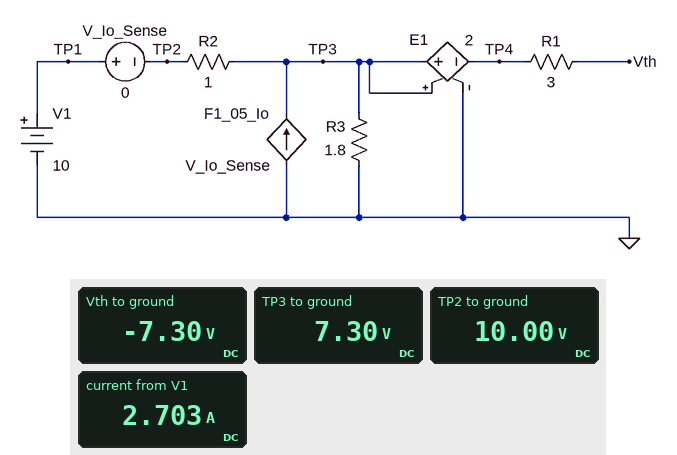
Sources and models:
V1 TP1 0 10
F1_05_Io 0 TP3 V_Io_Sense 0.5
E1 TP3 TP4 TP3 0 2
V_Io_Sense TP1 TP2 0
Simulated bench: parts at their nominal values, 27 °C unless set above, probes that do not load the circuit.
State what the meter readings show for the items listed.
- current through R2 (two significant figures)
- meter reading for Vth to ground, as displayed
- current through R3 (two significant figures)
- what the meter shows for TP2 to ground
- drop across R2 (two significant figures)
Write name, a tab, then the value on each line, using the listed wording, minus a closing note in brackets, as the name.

current through R2	2.7 A
meter reading for Vth to ground, as displayed	-7.30 V
current through R3	4.1 A
what the meter shows for TP2 to ground	10.00 V
drop across R2	2.7 V
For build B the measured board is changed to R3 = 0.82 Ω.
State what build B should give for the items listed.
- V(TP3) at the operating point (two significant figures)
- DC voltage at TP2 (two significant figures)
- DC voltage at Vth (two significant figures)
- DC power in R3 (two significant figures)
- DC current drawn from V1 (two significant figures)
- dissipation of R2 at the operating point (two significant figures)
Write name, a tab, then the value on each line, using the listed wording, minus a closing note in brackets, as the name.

V(TP3) at the operating point	5.5 V
DC voltage at TP2	10 V
DC voltage at Vth	-5.5 V
DC power in R3	37 W
DC current drawn from V1	4.5 A
dissipation of R2 at the operating point	20 W
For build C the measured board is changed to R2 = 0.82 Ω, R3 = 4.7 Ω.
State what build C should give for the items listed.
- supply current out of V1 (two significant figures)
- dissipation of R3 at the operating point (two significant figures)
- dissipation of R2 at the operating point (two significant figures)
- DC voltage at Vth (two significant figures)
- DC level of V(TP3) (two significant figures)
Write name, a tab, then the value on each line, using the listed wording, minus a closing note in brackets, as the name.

supply current out of V1	1.3 A
dissipation of R3 at the operating point	17 W
dissipation of R2 at the operating point	1.3 W
DC voltage at Vth	-9.0 V
DC level of V(TP3)	9.0 V
